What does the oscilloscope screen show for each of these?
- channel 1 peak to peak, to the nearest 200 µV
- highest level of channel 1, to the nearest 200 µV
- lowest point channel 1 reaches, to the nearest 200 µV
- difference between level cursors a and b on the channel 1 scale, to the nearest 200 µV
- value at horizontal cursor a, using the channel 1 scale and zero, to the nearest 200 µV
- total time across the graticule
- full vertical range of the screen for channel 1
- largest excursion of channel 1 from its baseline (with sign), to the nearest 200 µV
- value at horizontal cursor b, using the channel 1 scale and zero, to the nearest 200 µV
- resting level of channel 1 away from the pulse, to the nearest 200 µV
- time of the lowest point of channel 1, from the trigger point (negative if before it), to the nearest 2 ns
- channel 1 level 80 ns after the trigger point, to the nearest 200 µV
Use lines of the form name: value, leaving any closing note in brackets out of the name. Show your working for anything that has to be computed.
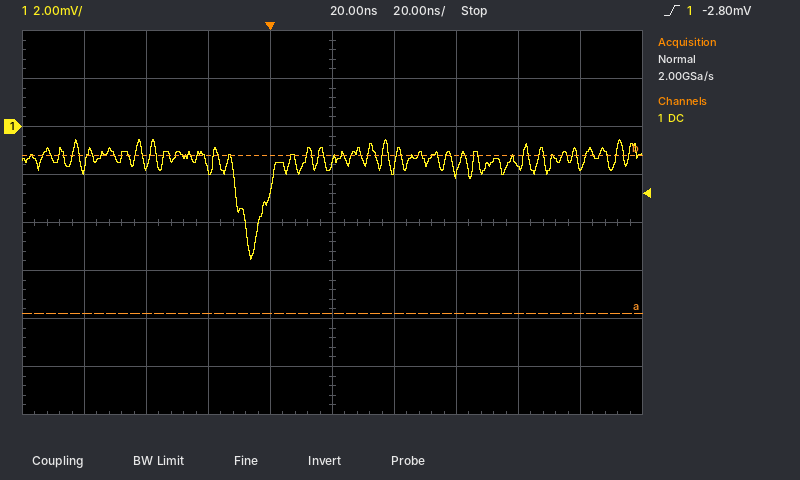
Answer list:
channel 1 peak to peak, to the nearest 200 µV: -600 µV − (-5.6 mV) = 5.0 mV
highest level of channel 1, to the nearest 200 µV: -600 µV
lowest point channel 1 reaches, to the nearest 200 µV: -5.6 mV
difference between level cursors a and b on the channel 1 scale, to the nearest 200 µV: 6.6 mV
value at horizontal cursor a, using the channel 1 scale and zero, to the nearest 200 µV: -7.8 mV
total time across the graticule: 200 ns
full vertical range of the screen for channel 1: 16 mV
largest excursion of channel 1 from its baseline (with sign), to the nearest 200 µV: -5.6 mV − (-1.4 mV) = -4.2 mV
value at horizontal cursor b, using the channel 1 scale and zero, to the nearest 200 µV: -1.2 mV
resting level of channel 1 away from the pulse, to the nearest 200 µV: -1.4 mV
time of the lowest point of channel 1, from the trigger point (negative if before it), to the nearest 2 ns: -6 ns
channel 1 level 80 ns after the trigger point, to the nearest 200 µV: -1.6 mV
